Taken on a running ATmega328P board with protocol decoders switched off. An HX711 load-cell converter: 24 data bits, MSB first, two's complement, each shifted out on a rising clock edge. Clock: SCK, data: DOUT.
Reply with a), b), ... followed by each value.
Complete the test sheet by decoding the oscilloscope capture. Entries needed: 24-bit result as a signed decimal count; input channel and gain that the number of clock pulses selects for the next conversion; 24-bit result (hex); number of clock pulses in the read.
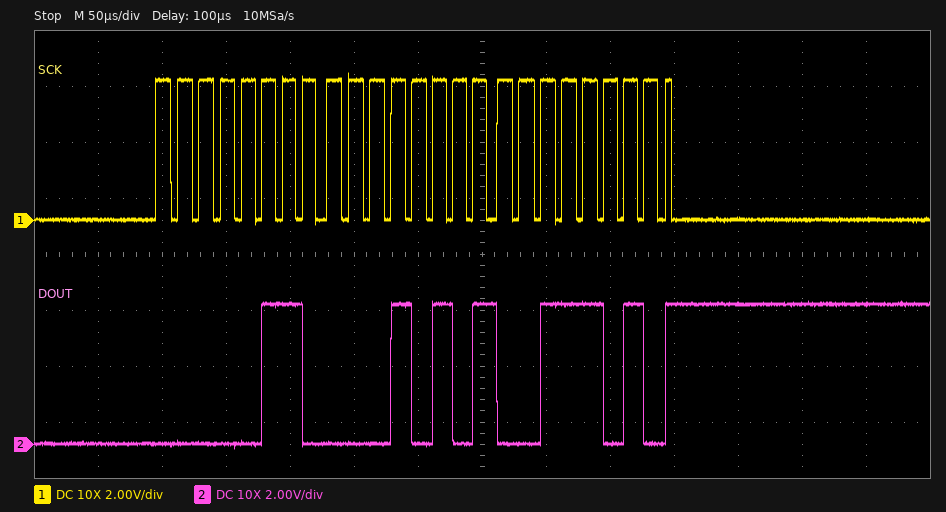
a) 398650
b) channel A, gain 128
c) 0x06153A
d) 25
